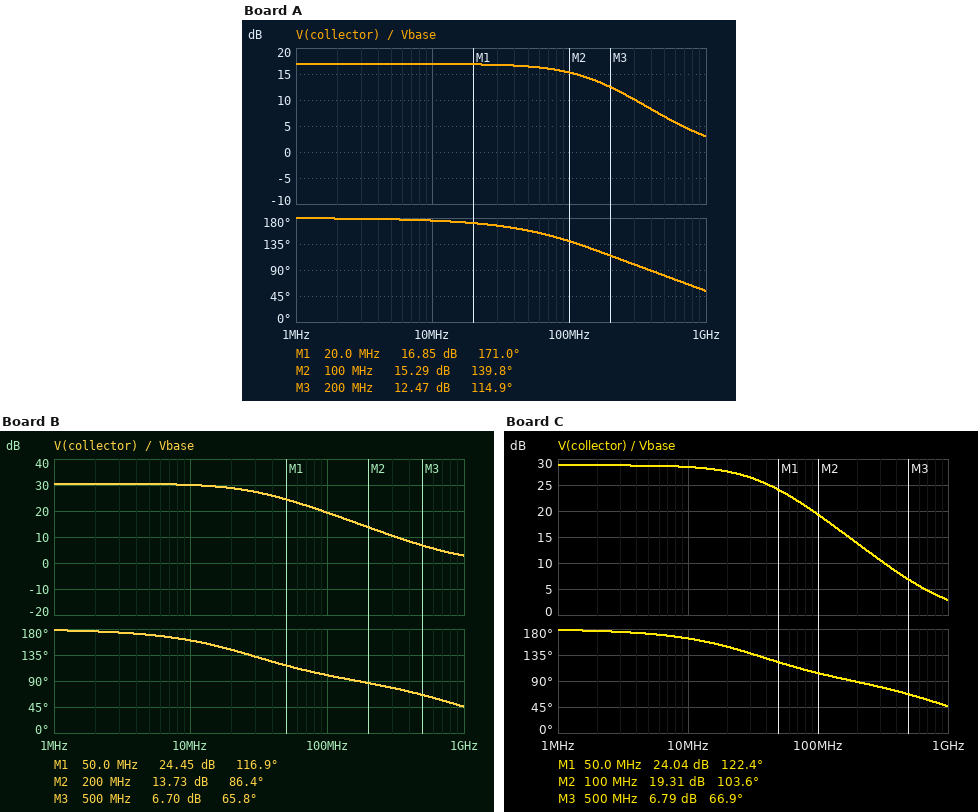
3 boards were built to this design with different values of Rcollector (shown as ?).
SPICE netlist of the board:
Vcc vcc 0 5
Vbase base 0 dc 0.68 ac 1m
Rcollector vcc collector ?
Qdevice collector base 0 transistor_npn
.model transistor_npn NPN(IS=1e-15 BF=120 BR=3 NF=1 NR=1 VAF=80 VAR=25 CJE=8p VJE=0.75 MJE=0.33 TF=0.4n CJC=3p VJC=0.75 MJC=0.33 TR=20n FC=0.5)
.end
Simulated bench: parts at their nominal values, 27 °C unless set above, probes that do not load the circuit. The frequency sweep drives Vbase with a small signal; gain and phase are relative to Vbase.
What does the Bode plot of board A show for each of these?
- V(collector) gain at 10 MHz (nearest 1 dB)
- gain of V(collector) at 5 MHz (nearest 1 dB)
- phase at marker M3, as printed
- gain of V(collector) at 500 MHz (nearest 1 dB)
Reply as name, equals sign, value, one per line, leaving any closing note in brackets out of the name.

V(collector) gain at 10 MHz = 17 dB
gain of V(collector) at 5 MHz = 17 dB
phase at marker M3, as printed = 114.9 deg
gain of V(collector) at 500 MHz = 7 dB
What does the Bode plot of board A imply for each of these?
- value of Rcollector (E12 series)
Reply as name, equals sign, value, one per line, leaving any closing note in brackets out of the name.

value of Rcollector = 680 Ω
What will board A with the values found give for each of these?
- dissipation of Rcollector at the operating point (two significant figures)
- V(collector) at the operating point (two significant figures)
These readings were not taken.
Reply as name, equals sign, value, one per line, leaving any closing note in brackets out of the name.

dissipation of Rcollector at the operating point = 49 µW
V(collector) at the operating point = 4.8 V
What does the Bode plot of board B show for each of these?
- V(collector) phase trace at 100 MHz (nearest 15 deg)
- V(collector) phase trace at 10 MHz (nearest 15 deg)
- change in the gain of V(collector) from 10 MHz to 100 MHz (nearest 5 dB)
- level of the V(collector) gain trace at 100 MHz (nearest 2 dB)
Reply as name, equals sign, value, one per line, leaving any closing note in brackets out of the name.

V(collector) phase trace at 100 MHz = 105 deg
V(collector) phase trace at 10 MHz = 165 deg
change in the gain of V(collector) from 10 MHz to 100 MHz = -10 dB
level of the V(collector) gain trace at 100 MHz = 20 dB
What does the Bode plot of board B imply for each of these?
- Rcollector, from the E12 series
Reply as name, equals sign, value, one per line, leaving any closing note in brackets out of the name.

Rcollector, from the E12 series = 3.3 kΩ
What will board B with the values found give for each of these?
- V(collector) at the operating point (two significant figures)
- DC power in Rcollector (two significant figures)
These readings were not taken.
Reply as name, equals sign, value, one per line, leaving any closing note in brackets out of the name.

V(collector) at the operating point = 4.1 V
DC power in Rcollector = 230 µW
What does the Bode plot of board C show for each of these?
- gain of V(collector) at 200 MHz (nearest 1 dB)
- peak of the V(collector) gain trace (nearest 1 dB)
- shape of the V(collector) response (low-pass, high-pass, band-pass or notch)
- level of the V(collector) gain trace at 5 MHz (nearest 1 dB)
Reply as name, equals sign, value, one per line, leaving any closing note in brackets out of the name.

gain of V(collector) at 200 MHz = 14 dB
peak of the V(collector) gain trace = 29 dB
shape of the V(collector) response = low-pass
level of the V(collector) gain trace at 5 MHz = 29 dB
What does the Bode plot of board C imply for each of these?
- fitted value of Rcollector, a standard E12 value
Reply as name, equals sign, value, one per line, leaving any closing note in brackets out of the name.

fitted value of Rcollector, a standard E12 value = 2.7 kΩ
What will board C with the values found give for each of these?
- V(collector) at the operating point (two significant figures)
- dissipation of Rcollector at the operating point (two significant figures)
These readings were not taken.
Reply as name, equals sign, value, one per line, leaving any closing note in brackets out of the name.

V(collector) at the operating point = 4.3 V
dissipation of Rcollector at the operating point = 190 µW
